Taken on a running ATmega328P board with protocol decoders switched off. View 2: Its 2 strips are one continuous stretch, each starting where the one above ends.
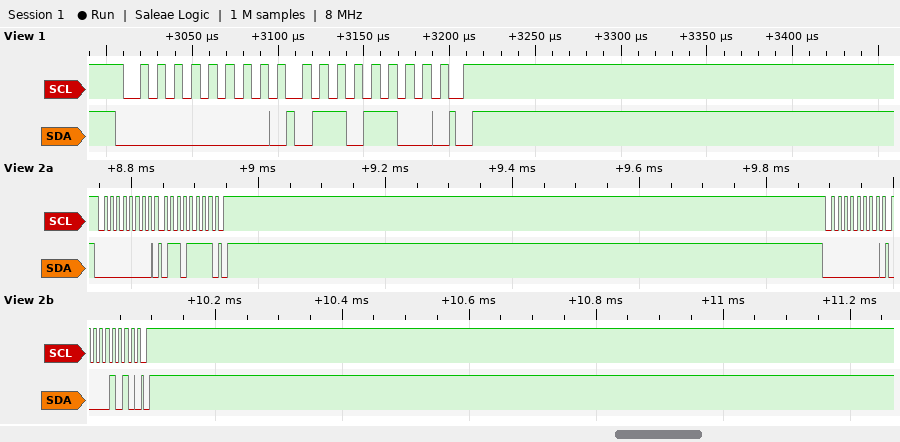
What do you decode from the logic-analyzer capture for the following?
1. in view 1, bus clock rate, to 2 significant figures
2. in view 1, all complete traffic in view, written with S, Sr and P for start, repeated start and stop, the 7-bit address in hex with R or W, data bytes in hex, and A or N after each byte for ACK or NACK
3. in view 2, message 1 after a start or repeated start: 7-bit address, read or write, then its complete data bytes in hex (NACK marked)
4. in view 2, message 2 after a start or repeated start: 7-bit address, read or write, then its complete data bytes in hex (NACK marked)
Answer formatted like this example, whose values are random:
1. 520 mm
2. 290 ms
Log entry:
1. 100 kHz
2. S 00W A 6C A P
3. 0x00 write: 6F
4. 0x00 write: 0A
